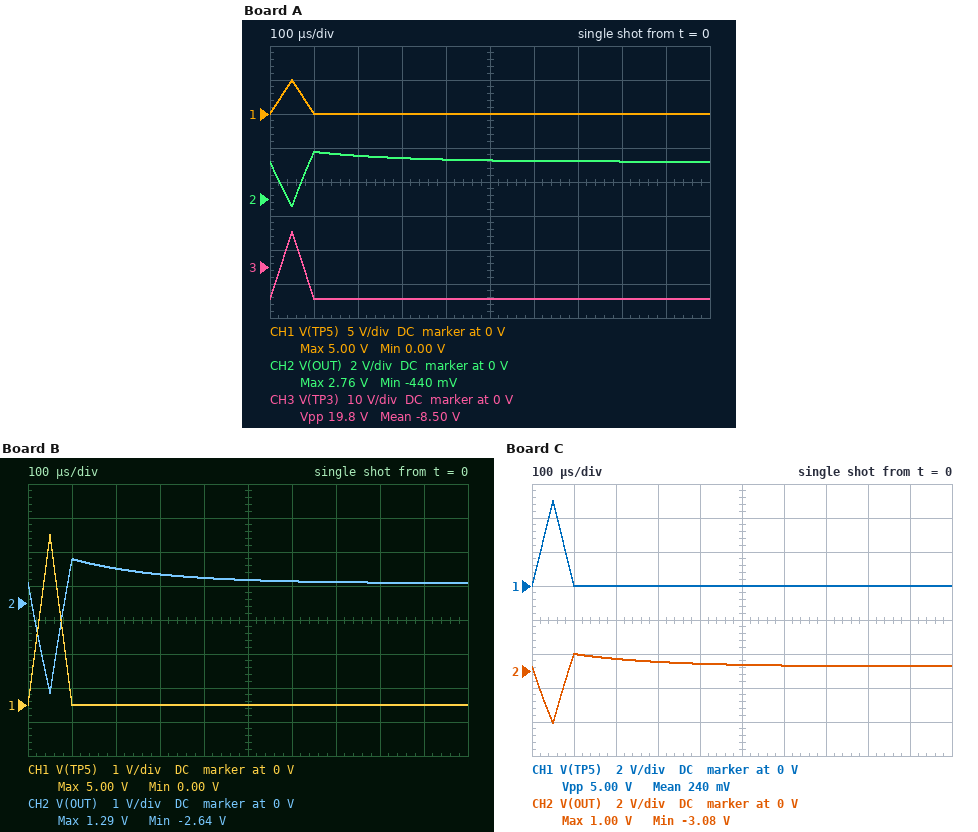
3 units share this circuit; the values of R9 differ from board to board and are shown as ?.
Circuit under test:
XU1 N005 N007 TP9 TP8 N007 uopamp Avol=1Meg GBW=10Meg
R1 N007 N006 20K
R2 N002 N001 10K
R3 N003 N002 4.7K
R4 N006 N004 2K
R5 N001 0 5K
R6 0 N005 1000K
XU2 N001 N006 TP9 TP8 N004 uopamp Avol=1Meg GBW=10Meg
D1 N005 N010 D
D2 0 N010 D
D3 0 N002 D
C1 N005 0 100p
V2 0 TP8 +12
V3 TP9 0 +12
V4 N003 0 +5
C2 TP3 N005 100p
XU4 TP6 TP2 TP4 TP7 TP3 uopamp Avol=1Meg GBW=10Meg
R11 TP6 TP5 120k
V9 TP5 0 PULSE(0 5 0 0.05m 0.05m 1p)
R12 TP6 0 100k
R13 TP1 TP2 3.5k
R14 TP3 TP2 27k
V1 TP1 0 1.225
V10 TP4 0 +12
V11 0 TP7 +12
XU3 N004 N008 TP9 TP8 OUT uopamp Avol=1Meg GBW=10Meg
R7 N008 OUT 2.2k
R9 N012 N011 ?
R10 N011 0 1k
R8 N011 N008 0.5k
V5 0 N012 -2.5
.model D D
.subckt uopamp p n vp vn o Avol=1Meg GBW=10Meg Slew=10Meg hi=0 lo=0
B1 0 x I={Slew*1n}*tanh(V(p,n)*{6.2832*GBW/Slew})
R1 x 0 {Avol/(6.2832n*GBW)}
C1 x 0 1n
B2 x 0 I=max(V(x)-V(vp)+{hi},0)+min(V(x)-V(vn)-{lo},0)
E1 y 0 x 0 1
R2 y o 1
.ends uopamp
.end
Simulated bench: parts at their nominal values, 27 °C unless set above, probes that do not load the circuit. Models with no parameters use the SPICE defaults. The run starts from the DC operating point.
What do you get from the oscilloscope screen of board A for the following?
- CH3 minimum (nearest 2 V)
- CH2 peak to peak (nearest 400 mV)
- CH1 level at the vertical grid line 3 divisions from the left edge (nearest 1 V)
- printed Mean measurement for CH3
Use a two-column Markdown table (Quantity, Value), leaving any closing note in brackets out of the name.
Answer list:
| Quantity | Value |
|---|---|
| CH3 minimum | -10 V |
| CH2 peak to peak | 3.2 V |
| CH1 level at the vertical grid line 3 divisions from the left edge | 0 V |
| printed Mean measurement for CH3 | -8.50 V |
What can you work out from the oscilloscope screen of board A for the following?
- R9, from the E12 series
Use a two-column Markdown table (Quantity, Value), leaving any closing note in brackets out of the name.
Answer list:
| Quantity | Value |
|---|---|
| R9, from the E12 series | 1.5 kΩ |
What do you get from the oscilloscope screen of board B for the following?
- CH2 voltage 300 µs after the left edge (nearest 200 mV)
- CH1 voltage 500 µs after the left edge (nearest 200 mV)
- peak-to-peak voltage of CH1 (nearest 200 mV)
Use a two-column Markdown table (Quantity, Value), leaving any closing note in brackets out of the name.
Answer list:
| Quantity | Value |
|---|---|
| CH2 voltage 300 µs after the left edge | 800 mV |
| CH1 voltage 500 µs after the left edge | 0 V |
| peak-to-peak voltage of CH1 | 5.0 V |
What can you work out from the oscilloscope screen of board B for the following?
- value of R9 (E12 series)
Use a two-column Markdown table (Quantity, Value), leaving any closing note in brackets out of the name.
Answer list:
| Quantity | Value |
|---|---|
| value of R9 | 470 Ω |
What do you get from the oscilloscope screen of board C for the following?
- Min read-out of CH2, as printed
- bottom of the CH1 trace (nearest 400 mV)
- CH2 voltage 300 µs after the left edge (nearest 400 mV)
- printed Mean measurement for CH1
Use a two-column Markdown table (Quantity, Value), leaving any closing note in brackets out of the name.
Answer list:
| Quantity | Value |
|---|---|
| Min read-out of CH2, as printed | -3.08 V |
| bottom of the CH1 trace | 0 V |
| CH2 voltage 300 µs after the left edge | 400 mV |
| printed Mean measurement for CH1 | 240 mV |
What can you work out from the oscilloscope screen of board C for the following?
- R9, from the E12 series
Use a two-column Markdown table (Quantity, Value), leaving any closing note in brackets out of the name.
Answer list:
| Quantity | Value |
|---|---|
| R9, from the E12 series | 390 Ω |
